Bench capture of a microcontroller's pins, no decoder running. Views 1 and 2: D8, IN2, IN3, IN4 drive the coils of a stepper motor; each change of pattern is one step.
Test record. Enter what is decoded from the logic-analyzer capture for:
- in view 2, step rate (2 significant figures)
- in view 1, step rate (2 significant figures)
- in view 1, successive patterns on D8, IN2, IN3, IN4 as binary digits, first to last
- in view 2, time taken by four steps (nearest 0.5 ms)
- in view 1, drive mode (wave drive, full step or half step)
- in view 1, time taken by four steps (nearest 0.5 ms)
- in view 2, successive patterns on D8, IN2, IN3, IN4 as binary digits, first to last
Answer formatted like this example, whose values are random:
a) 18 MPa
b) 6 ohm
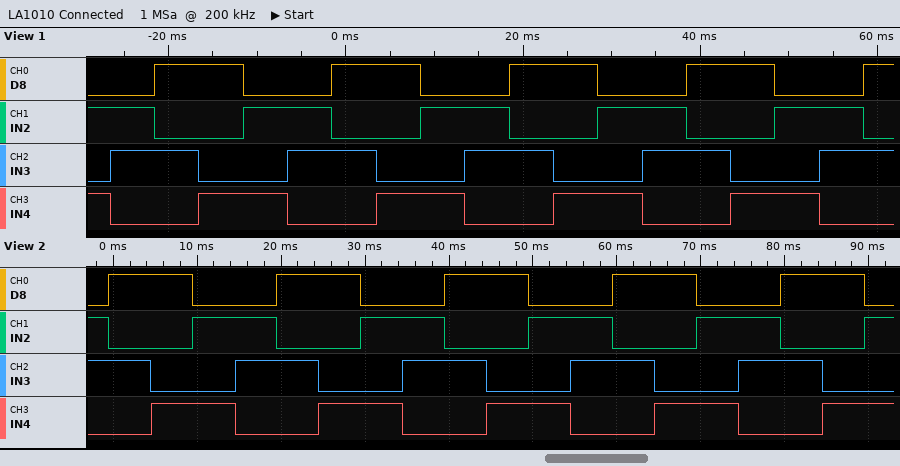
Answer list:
a) 200 steps/s
b) 200 steps/s
c) 0101 0110 1010 1001 0101 0110 1010 1001 0101 0110 1010 1001 0101 0110 1010 1001 0101 0110 1010
d) 20.0 ms
e) full step
f) 20.0 ms
g) 0110 1010 1001 0101 0110 1010 1001 0101 0110 1010 1001 0101 0110 1010 1001 0101 0110 1010 1001 0101
